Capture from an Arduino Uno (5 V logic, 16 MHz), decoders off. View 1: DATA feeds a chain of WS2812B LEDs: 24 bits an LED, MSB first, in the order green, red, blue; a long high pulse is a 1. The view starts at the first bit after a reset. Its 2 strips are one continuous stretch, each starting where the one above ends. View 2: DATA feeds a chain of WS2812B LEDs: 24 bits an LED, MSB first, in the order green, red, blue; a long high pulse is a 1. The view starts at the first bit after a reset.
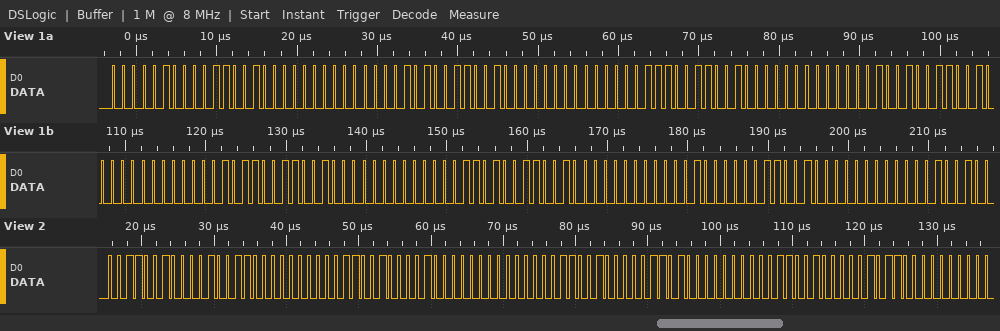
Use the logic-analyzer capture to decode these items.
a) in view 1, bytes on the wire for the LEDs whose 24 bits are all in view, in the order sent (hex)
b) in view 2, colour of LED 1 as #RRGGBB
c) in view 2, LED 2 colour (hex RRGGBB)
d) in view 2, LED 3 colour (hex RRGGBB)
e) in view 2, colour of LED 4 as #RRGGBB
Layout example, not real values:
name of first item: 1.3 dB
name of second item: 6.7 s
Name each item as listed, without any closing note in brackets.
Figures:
in view 1, bytes on the wire for the LEDs whose 24 bits are all in view, in the order sent: 04 32 00 05 32 00 07 32 00 09 32 00 0B 32 00 0D 32 00 10 32 00
in view 2, colour of LED 1 as #RRGGBB: #133200
in view 2, LED 2 colour: #103200
in view 2, LED 3 colour: #0D3200
in view 2, colour of LED 4 as #RRGGBB: #0B3200
